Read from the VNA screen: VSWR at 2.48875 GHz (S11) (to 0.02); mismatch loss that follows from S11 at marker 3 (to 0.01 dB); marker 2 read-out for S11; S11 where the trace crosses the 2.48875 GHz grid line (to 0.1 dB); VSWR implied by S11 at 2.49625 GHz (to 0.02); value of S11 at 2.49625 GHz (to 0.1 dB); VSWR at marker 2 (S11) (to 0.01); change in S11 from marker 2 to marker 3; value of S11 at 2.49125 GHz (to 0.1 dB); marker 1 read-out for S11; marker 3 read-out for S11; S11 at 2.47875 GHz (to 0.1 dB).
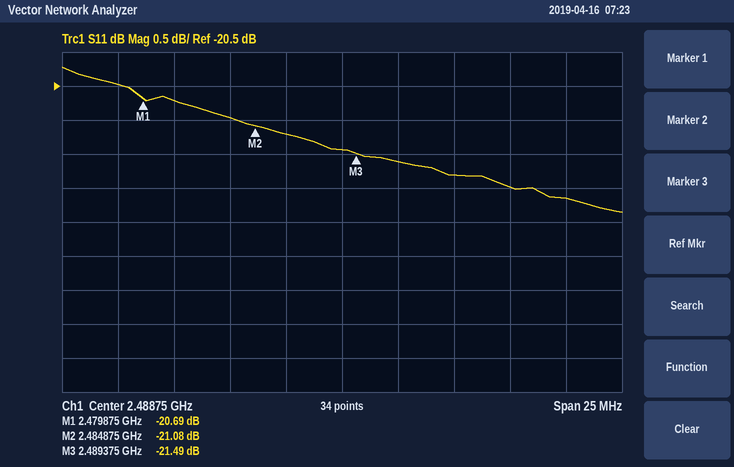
1.18
0.03 dB
-21.08 dB
-21.4 dB
1.18
-22.0 dB
1.19
-0.41 dB
-21.6 dB
-20.69 dB
-21.49 dB
-20.5 dB
